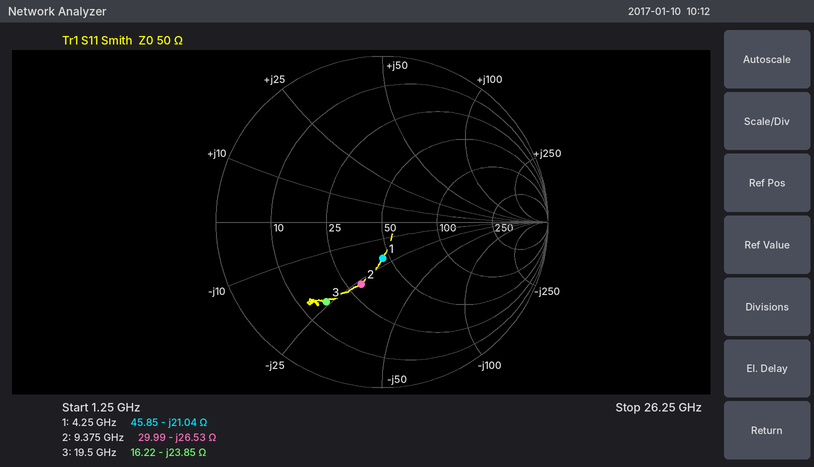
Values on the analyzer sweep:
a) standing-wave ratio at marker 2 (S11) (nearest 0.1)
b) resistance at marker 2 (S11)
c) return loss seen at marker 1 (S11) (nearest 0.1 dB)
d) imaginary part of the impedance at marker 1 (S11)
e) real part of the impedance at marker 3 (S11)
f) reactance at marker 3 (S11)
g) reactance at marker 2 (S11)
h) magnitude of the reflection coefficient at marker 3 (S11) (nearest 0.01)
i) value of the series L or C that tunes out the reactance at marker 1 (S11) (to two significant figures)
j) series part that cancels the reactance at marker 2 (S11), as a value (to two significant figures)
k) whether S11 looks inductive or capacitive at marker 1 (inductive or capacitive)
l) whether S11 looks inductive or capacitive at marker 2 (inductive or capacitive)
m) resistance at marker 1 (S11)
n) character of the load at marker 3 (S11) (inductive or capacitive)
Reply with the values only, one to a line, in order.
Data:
2.3
29.99 Ω
13.2 dB
-21.04 Ω
16.22 Ω
-23.85 Ω
-26.53 Ω
0.59
790 pH
450 pH
capacitive
capacitive
45.85 Ω
capacitive
